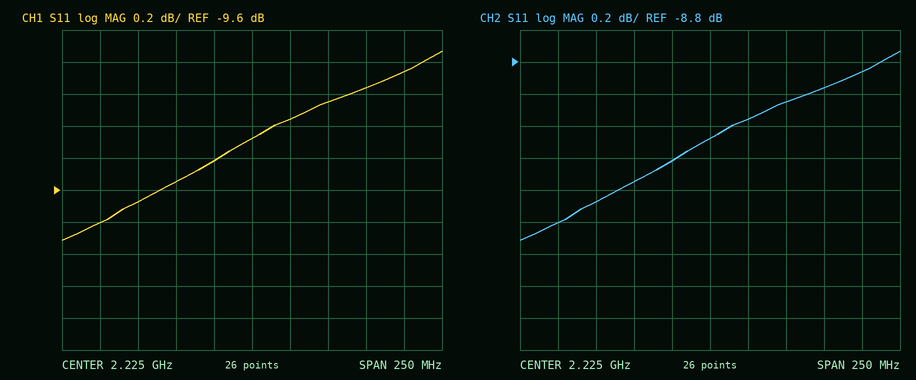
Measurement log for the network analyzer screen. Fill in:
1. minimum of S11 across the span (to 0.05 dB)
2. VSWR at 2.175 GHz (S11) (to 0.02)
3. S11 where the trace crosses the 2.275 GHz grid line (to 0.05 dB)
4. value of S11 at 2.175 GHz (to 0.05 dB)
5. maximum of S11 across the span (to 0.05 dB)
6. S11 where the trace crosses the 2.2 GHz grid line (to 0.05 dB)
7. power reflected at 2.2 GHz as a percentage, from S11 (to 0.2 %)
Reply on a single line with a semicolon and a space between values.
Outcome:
-9.90 dB; 2.00; -9.05 dB; -9.55 dB; -8.75 dB; -9.40 dB; 11.4 %
